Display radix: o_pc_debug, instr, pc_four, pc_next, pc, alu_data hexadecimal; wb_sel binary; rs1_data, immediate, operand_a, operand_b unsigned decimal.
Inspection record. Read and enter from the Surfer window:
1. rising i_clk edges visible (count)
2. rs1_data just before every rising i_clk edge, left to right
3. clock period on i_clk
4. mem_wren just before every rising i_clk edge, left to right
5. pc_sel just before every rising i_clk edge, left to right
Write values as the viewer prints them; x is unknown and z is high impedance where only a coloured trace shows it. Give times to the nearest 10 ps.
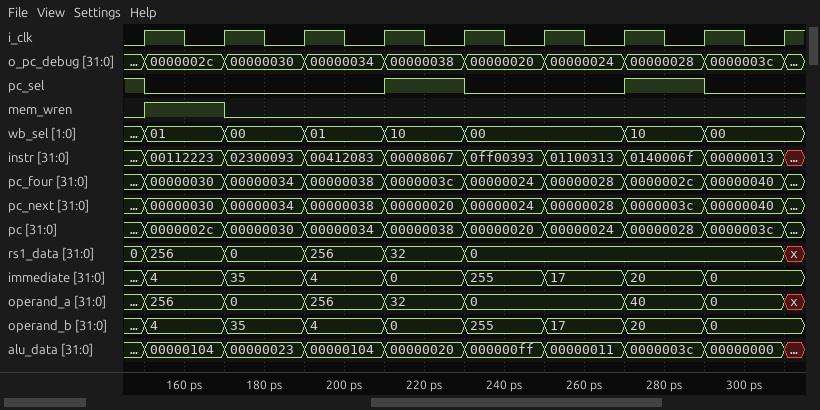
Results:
9
0, 256, 0, 256, 32, 0, 0, 0, 0
20 ps
0 1 0 0 0 0 0 0 0
1 0 0 0 1 0 0 1 0
